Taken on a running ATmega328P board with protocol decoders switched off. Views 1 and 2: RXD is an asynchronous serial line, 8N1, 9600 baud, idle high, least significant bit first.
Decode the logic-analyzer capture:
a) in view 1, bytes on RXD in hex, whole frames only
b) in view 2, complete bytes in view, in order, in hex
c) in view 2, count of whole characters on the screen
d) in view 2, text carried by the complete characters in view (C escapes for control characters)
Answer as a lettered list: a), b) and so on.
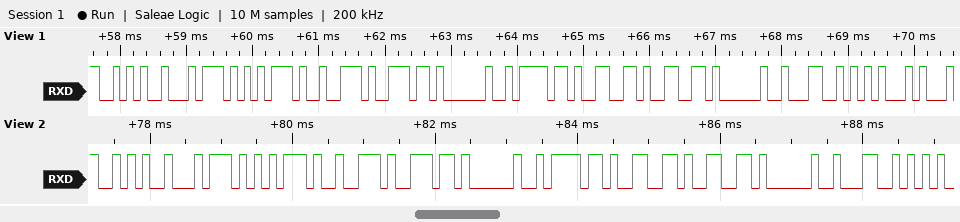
a) 2A 74 75 72 6E 20 6F 66 66 20 4C 45
b) 2A 74 75 72 6E 20 6F 66 66 20 4C
c) 11
d) "*turn off L"
